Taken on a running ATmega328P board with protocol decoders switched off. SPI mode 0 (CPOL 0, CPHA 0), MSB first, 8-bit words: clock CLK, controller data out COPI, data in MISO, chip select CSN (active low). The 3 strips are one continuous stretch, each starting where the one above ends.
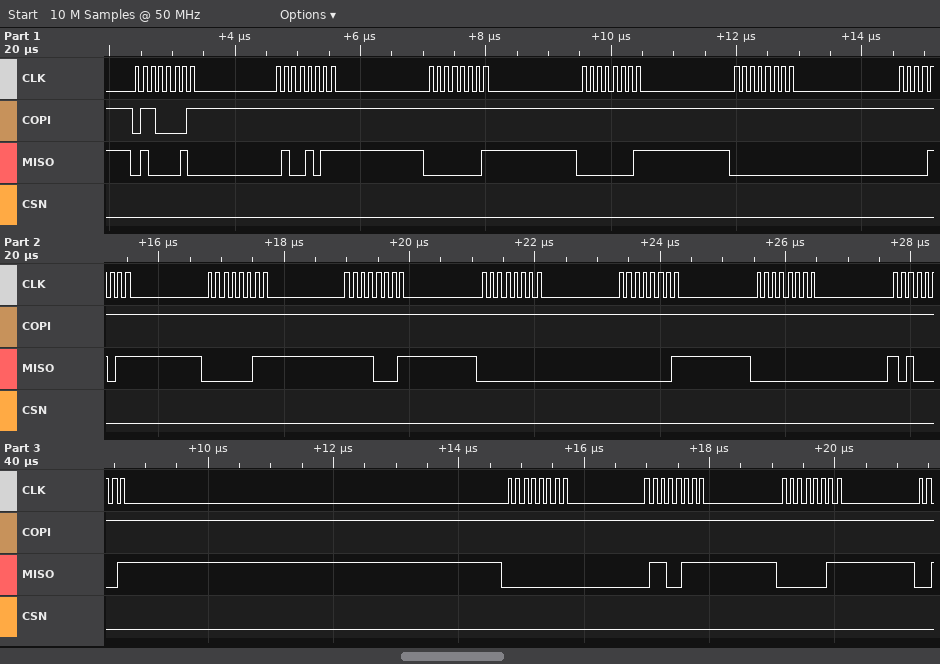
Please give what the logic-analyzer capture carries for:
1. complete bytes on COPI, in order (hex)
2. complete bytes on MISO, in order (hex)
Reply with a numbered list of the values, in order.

1. 61 FF FF FF FF FF FF FF FF FF FF FF FF FF FF
2. 42 4B 01 01 00 0B 03 F1 00 01 00 A1 00 67 03
